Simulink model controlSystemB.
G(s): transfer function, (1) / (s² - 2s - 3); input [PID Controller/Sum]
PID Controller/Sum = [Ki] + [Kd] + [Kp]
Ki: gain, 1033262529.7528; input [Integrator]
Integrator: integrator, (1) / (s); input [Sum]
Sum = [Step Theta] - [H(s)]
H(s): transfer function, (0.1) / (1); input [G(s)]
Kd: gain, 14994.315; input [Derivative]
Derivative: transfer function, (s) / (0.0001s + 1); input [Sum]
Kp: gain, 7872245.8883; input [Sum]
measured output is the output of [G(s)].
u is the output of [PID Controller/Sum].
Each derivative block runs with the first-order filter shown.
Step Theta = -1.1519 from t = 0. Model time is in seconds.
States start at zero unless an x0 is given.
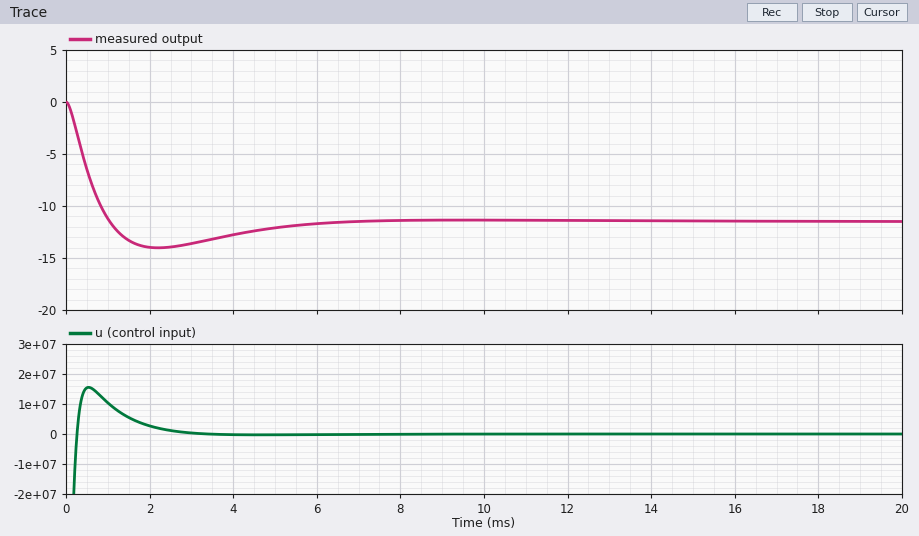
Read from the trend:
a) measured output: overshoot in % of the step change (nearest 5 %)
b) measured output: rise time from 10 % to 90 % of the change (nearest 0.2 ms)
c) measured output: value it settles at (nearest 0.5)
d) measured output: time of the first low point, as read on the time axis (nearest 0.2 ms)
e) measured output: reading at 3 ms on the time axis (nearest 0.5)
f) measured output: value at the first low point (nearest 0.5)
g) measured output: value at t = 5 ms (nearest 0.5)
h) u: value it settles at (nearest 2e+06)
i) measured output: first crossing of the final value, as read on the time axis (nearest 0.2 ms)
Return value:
20 %
0.8 ms
-11.5
2.2 ms
-13.5
-14.0
-12.0
0
1.0 ms
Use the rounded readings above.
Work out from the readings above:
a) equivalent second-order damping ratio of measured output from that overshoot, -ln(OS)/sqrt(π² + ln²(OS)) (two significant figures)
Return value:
0.46
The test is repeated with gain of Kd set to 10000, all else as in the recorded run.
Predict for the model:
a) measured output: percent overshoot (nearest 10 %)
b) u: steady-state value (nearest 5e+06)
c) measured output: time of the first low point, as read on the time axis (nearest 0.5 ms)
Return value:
30 %
0
2.5 ms
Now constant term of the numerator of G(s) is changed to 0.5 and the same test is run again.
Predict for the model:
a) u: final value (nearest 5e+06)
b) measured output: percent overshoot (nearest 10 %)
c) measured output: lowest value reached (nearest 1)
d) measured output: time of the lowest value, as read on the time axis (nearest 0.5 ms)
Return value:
0
30 %
-15
3.5 ms
